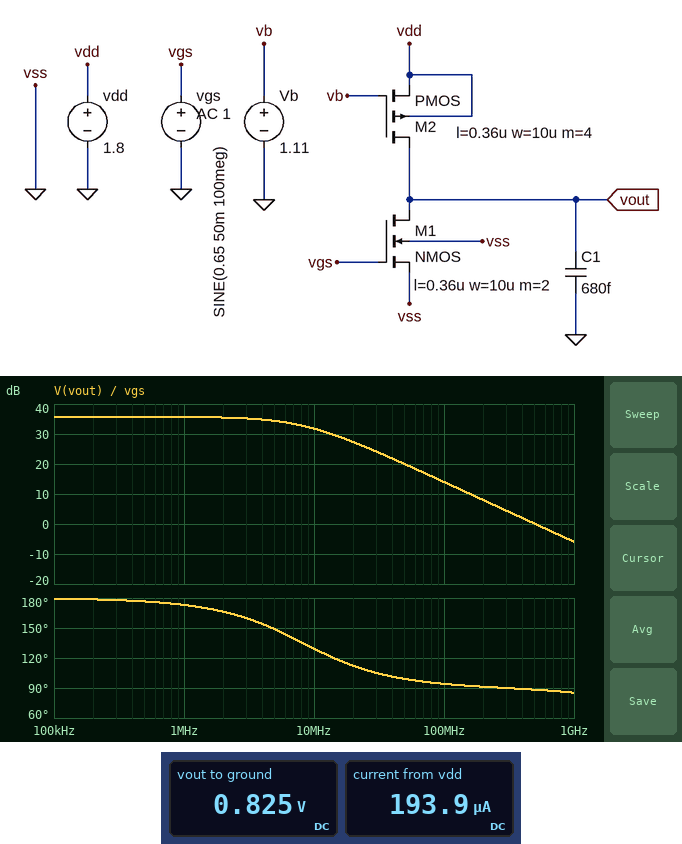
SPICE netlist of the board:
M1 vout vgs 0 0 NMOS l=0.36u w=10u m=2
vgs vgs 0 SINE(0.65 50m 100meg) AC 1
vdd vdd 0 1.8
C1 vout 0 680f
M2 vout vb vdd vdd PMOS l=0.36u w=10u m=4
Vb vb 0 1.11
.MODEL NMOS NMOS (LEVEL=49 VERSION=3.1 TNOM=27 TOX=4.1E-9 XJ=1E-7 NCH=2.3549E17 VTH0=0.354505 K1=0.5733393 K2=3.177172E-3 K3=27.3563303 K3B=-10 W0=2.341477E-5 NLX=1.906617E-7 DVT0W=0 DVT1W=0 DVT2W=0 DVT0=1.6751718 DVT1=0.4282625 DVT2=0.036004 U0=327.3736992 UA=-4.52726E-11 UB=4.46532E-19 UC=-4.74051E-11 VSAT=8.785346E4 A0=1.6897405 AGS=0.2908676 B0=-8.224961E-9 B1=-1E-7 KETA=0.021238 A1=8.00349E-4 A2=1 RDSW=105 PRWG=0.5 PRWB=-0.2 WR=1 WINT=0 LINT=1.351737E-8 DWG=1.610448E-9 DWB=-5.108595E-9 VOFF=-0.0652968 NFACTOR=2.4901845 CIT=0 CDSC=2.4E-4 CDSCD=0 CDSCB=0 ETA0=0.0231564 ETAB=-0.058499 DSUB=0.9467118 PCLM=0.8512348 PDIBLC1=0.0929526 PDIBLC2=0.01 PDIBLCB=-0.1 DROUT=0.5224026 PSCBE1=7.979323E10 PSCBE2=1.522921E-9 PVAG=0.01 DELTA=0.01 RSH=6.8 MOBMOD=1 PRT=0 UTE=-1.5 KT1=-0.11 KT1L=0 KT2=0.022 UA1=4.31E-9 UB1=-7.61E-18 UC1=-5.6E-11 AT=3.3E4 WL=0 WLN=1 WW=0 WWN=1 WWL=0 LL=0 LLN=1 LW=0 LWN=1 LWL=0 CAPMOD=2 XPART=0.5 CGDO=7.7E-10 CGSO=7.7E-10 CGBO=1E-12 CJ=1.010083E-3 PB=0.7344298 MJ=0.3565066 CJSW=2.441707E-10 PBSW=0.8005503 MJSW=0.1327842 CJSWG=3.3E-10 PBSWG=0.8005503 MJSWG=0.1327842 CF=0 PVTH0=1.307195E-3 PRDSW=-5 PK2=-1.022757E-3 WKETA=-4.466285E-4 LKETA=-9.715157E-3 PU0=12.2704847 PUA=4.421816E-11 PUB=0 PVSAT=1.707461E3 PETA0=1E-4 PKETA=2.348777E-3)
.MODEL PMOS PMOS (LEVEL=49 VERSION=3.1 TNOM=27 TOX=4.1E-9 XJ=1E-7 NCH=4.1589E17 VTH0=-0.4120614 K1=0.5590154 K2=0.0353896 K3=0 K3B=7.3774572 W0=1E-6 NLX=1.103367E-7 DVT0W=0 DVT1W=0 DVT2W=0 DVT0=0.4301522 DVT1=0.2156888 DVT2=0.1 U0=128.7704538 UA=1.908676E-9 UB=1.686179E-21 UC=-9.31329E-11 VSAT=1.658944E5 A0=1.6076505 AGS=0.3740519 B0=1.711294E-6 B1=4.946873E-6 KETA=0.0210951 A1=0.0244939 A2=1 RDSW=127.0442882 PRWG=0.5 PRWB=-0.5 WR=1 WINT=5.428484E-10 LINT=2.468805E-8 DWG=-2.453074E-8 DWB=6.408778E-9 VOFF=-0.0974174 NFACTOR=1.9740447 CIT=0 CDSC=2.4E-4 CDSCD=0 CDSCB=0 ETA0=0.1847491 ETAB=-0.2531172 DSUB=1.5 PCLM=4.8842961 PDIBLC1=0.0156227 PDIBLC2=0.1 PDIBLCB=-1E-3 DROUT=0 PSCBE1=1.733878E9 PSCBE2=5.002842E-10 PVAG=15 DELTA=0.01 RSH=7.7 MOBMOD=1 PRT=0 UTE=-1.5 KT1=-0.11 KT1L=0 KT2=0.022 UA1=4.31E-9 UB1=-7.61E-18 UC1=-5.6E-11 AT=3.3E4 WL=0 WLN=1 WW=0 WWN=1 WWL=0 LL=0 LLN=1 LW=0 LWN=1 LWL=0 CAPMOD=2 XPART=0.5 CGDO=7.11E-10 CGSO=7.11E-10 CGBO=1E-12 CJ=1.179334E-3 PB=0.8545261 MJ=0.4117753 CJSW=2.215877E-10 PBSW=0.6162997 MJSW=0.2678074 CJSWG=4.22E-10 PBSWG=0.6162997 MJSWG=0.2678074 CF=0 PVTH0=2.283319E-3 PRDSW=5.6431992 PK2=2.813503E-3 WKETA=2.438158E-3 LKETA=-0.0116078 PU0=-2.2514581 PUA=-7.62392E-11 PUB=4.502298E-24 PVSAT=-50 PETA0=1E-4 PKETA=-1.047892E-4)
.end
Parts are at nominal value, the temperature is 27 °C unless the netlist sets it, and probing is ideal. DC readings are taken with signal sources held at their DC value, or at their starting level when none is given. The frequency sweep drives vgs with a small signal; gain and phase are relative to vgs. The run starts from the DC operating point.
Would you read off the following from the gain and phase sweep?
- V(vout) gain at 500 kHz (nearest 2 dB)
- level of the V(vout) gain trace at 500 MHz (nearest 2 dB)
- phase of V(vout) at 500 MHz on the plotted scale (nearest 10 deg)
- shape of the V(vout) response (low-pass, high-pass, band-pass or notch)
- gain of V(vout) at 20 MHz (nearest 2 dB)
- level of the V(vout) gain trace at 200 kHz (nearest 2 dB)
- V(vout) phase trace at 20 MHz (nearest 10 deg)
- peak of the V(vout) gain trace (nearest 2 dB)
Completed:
36 dB
0 dB
90 deg
low-pass
28 dB
36 dB
110 deg
36 dB
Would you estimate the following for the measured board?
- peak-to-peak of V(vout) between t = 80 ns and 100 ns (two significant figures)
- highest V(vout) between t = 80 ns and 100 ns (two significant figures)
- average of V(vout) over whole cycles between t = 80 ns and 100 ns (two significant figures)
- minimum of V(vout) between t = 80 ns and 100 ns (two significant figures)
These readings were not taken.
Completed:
490 mV
840 mV
600 mV
350 mV
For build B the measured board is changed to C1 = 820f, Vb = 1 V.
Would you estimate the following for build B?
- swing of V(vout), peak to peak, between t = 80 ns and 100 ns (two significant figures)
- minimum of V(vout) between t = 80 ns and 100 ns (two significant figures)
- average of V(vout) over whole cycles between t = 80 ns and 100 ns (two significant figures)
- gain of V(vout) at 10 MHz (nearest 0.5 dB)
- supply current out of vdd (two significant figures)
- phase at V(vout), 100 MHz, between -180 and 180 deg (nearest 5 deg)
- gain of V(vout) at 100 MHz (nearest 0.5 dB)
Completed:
150 mV
1.6 V
1.7 V
3.0 dB
210 µA
160 deg
2.5 dB
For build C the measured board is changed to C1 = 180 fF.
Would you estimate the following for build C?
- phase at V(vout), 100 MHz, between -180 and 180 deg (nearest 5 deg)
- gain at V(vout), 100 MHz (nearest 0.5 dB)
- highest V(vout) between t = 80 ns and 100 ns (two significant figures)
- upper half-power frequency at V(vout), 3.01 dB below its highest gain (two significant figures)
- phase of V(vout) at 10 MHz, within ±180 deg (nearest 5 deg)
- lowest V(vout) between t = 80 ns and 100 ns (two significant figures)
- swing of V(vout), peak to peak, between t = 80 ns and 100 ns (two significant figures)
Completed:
105 deg
23.5 dB
1.5 V
25 MHz
160 deg
110 mV
1.4 V
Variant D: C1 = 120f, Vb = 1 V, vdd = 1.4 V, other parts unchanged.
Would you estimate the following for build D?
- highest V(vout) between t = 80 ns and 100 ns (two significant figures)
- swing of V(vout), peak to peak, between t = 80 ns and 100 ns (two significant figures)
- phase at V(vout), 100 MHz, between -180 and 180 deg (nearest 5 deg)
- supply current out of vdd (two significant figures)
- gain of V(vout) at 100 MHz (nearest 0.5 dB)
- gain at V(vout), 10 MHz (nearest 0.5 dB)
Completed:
1.6 mV
1.4 mV
110 deg
1.7 µA
-37.5 dB
-45.0 dB
